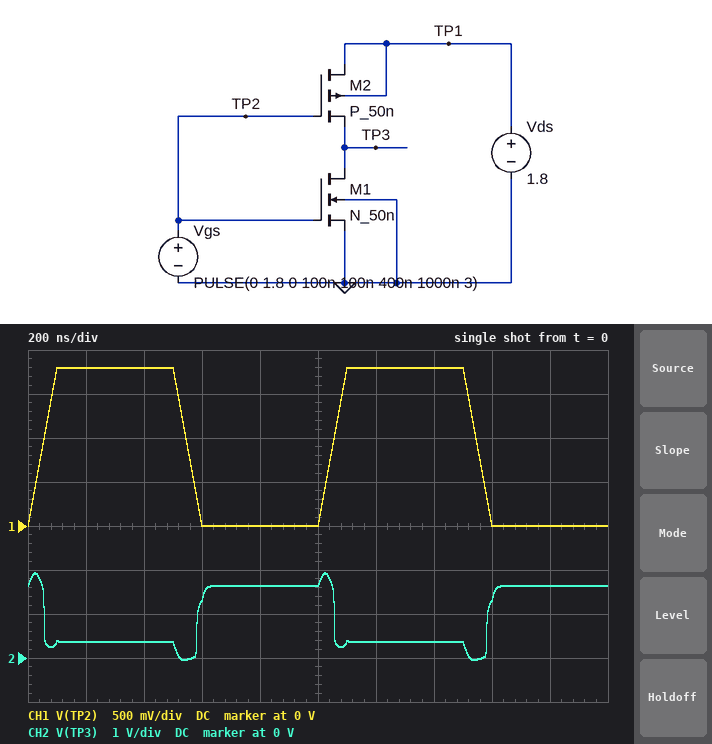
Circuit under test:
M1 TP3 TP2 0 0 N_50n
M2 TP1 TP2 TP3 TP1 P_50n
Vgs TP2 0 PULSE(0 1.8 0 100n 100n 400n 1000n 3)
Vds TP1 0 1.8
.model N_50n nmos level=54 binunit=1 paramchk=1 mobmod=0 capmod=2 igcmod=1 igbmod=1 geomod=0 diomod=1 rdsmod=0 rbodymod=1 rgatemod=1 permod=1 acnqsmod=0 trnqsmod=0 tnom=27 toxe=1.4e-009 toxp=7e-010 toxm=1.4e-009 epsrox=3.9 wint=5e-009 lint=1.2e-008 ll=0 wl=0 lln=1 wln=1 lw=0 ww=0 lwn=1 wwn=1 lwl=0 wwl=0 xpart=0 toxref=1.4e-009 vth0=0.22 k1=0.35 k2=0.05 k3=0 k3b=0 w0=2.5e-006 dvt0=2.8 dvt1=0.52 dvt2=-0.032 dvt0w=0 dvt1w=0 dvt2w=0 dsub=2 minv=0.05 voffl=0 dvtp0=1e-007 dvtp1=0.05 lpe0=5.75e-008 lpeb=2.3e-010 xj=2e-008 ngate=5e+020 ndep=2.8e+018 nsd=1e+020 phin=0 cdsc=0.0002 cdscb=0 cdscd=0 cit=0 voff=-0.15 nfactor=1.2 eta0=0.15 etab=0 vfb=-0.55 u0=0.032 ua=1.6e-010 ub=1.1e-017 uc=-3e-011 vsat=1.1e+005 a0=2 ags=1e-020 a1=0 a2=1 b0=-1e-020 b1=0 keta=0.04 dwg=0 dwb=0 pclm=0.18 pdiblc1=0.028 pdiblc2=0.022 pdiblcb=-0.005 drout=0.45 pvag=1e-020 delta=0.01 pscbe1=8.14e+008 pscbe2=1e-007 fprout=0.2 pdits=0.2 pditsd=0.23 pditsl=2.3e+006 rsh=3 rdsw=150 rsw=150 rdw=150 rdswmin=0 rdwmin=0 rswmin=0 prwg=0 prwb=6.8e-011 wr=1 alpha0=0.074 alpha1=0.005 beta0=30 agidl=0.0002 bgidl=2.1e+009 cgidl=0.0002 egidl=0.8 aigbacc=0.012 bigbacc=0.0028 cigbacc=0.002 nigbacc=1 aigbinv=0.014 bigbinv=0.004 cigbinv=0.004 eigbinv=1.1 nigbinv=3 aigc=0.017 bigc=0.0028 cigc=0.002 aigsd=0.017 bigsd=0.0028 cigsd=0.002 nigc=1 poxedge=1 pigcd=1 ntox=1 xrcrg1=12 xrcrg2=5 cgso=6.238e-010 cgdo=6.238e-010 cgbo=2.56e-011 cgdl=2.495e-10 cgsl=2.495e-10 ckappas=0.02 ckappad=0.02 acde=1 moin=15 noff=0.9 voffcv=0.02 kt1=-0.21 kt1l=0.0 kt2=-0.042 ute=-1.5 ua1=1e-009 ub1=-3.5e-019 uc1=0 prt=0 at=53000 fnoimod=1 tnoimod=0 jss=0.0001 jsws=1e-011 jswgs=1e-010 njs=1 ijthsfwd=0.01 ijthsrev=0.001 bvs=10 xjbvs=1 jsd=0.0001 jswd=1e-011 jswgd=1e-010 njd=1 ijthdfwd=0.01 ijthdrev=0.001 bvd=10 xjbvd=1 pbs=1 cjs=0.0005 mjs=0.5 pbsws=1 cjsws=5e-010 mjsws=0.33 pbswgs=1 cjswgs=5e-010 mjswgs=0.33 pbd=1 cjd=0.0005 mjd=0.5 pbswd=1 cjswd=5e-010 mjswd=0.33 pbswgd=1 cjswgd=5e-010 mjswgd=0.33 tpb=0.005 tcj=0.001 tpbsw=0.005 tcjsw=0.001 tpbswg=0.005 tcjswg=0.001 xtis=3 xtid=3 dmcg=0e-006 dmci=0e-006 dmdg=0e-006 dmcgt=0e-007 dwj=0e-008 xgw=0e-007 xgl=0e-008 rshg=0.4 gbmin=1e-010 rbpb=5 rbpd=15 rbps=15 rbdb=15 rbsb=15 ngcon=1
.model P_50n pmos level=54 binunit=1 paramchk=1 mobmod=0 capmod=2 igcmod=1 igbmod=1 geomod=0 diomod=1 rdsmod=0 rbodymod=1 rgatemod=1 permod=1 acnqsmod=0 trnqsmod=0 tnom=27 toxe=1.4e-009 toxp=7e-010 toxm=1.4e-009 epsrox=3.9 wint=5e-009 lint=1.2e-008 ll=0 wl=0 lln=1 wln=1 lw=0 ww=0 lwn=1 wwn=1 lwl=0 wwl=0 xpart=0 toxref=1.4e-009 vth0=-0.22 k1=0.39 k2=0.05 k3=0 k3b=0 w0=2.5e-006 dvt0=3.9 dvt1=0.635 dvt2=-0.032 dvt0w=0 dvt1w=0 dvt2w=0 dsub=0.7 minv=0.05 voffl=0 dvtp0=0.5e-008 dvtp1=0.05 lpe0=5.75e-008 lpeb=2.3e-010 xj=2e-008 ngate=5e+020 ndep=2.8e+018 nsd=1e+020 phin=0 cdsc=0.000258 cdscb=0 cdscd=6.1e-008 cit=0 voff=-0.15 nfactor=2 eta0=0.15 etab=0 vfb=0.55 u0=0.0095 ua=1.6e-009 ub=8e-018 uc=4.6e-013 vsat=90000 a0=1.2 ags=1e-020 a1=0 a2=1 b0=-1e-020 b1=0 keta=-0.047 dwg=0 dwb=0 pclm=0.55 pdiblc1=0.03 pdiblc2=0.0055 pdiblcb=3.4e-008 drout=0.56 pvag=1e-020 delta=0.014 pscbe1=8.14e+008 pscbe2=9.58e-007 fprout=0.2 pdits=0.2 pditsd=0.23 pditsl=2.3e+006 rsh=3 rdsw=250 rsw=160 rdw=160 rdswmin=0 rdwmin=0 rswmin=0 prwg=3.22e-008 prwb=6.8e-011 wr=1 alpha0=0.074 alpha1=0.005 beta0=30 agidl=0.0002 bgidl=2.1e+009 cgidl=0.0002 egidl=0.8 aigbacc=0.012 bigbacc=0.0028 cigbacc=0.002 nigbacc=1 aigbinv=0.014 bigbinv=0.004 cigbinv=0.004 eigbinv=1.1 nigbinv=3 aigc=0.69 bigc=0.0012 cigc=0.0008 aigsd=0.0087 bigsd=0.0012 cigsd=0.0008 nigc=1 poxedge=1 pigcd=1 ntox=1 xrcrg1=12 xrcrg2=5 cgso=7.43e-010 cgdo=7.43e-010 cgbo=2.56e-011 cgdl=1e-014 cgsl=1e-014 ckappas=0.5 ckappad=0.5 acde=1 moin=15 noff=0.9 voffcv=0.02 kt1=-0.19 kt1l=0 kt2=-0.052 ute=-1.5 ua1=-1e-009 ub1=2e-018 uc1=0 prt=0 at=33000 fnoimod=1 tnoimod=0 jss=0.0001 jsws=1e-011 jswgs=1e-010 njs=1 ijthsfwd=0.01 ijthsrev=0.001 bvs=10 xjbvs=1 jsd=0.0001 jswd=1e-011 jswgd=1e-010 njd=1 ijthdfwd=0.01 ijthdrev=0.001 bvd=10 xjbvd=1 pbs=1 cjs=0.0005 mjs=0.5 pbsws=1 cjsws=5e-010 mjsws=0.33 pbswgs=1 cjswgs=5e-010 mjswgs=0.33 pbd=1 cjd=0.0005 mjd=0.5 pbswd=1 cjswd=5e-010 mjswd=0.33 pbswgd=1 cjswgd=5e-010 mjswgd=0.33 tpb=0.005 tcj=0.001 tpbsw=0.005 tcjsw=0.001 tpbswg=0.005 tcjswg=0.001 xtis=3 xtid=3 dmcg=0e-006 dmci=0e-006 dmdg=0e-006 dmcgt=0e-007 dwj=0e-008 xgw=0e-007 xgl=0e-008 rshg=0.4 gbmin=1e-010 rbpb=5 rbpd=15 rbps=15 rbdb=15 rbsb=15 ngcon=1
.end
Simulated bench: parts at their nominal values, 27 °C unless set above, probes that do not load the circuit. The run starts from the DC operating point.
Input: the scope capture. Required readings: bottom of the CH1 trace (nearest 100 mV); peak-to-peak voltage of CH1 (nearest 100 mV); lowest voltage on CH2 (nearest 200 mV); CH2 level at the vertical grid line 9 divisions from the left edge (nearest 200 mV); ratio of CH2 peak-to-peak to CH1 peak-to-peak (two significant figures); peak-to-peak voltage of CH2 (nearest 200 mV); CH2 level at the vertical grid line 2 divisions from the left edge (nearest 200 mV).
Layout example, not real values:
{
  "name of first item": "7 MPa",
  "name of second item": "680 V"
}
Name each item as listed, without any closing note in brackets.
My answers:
{
  "bottom of the CH1 trace": "0 V",
  "peak-to-peak voltage of CH1": "1.8 V",
  "lowest voltage on CH2": "0 V",
  "CH2 level at the vertical grid line 9 divisions from the left edge": "1.6 V",
  "ratio of CH2 peak-to-peak to CH1 peak-to-peak": "1.1",
  "peak-to-peak voltage of CH2": "2.0 V",
  "CH2 level at the vertical grid line 2 divisions from the left edge": "400 mV"
}
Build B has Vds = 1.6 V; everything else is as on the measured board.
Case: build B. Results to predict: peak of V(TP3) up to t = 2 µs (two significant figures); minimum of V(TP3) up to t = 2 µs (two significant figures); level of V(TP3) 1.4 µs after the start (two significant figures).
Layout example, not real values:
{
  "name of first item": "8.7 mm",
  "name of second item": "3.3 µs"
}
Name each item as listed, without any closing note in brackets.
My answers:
{
  "peak of V(TP3) up to t = 2 µs": "1.8 V",
  "minimum of V(TP3) up to t = 2 µs": "-72 mV",
  "level of V(TP3) 1.4 µs after the start": "370 mV"
}
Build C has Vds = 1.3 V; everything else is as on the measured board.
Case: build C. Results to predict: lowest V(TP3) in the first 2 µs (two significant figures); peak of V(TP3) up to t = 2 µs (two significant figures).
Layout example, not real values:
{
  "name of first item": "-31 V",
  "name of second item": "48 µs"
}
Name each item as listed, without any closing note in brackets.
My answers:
{
  "lowest V(TP3) in the first 2 µs": "-95 mV",
  "peak of V(TP3) up to t = 2 µs": "1.5 V"
}
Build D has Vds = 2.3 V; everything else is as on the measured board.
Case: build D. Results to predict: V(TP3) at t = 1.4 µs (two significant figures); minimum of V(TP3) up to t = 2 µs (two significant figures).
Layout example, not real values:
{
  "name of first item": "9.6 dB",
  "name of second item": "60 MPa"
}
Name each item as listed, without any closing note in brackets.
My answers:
{
  "V(TP3) at t = 1.4 µs": "420 mV",
  "minimum of V(TP3) up to t = 2 µs": "22 mV"
}
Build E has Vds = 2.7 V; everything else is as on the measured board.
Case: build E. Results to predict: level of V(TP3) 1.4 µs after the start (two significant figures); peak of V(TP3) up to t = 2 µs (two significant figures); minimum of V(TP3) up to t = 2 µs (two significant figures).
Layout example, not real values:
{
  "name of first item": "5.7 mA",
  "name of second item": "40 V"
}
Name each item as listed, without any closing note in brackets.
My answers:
{
  "level of V(TP3) 1.4 µs after the start": "520 mV",
  "peak of V(TP3) up to t = 2 µs": "2.3 V",
  "minimum of V(TP3) up to t = 2 µs": "69 mV"
}
